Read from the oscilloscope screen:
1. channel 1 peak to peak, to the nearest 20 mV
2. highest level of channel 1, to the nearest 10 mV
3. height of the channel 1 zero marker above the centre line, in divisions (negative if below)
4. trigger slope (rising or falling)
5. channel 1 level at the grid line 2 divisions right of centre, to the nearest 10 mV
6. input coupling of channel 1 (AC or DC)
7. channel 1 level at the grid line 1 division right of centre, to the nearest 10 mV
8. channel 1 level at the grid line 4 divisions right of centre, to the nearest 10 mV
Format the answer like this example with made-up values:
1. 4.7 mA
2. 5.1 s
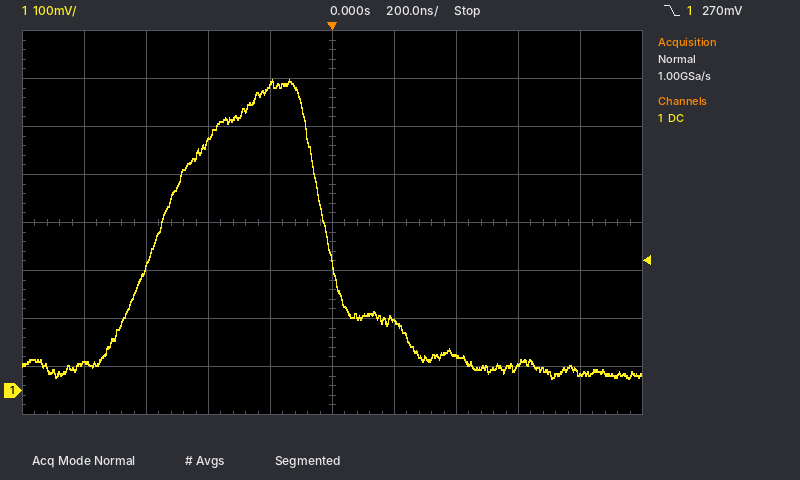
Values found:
1. 620 mV
2. 650 mV
3. -3.5 div
4. falling
5. 70 mV
6. DC
7. 150 mV
8. 40 mV
